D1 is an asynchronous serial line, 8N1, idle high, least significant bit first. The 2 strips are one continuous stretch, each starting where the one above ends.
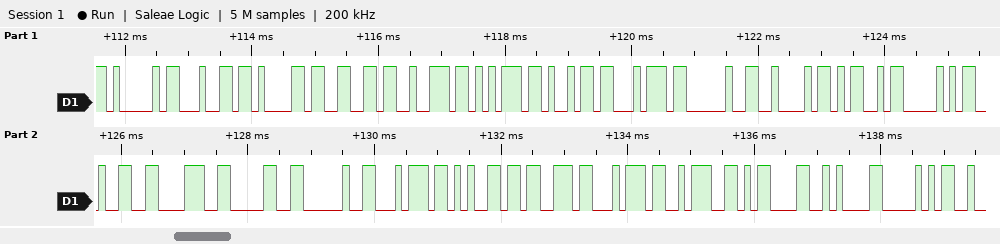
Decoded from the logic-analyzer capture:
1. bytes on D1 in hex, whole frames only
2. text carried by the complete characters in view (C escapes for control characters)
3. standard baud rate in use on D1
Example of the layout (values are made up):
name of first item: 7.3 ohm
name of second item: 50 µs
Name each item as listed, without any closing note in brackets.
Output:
bytes on D1 in hex, whole frames only: 41 64 61 66 72 75 69 74 20 42 4D 50 32 38 30 20 74 65 73 74 3A 0D 0A 50
text carried by the complete characters in view: "Adafruit BMP280 test:\r\nP"
standard baud rate in use on D1: 9600 baud
